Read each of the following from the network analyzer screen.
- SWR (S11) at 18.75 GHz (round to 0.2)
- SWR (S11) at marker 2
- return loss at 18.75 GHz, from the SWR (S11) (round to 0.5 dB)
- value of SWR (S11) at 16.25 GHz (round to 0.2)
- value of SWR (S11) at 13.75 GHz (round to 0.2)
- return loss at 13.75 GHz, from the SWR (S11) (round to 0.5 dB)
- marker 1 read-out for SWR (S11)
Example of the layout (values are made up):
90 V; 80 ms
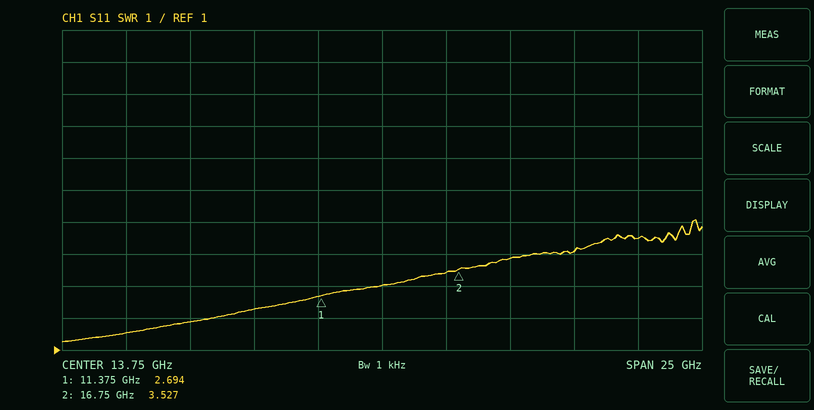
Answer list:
3.8; 3.527; 4.5 dB; 3.4; 3.0; 6.0 dB; 2.694
